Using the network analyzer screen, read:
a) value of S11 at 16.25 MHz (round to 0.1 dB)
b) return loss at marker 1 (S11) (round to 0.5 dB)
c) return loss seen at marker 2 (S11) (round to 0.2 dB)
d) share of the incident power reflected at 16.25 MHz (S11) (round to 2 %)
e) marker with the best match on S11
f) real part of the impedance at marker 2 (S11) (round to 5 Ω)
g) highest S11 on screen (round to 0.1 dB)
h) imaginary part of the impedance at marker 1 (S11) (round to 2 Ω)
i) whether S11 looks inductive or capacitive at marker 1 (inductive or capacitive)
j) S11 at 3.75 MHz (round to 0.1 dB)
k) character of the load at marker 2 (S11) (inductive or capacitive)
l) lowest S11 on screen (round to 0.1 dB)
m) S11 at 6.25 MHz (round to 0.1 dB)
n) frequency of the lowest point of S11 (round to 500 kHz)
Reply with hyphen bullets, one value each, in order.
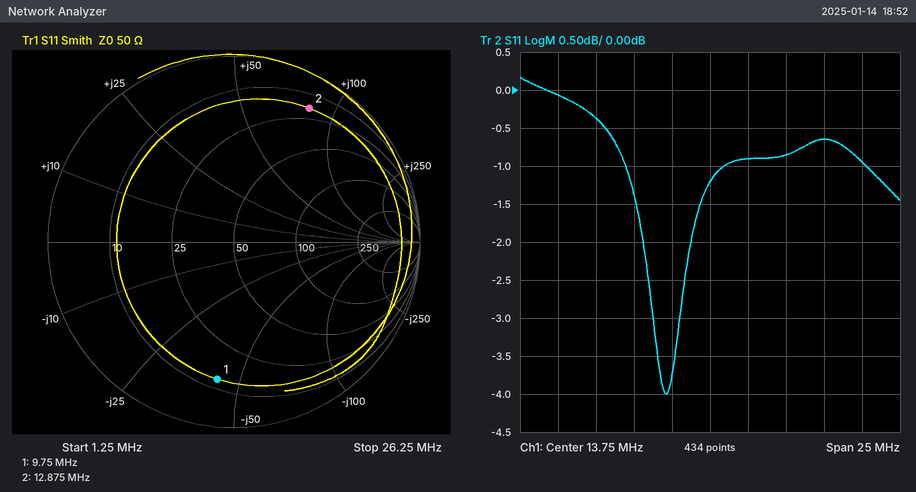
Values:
- -0.9 dB
- 2.5 dB
- 1.6 dB
- 82 %
- marker 1
- 20 Ω
- 0.2 dB
- -42 Ω
- capacitive
- -0.1 dB
- inductive
- -4.0 dB
- -0.4 dB
- 11.0 MHz
